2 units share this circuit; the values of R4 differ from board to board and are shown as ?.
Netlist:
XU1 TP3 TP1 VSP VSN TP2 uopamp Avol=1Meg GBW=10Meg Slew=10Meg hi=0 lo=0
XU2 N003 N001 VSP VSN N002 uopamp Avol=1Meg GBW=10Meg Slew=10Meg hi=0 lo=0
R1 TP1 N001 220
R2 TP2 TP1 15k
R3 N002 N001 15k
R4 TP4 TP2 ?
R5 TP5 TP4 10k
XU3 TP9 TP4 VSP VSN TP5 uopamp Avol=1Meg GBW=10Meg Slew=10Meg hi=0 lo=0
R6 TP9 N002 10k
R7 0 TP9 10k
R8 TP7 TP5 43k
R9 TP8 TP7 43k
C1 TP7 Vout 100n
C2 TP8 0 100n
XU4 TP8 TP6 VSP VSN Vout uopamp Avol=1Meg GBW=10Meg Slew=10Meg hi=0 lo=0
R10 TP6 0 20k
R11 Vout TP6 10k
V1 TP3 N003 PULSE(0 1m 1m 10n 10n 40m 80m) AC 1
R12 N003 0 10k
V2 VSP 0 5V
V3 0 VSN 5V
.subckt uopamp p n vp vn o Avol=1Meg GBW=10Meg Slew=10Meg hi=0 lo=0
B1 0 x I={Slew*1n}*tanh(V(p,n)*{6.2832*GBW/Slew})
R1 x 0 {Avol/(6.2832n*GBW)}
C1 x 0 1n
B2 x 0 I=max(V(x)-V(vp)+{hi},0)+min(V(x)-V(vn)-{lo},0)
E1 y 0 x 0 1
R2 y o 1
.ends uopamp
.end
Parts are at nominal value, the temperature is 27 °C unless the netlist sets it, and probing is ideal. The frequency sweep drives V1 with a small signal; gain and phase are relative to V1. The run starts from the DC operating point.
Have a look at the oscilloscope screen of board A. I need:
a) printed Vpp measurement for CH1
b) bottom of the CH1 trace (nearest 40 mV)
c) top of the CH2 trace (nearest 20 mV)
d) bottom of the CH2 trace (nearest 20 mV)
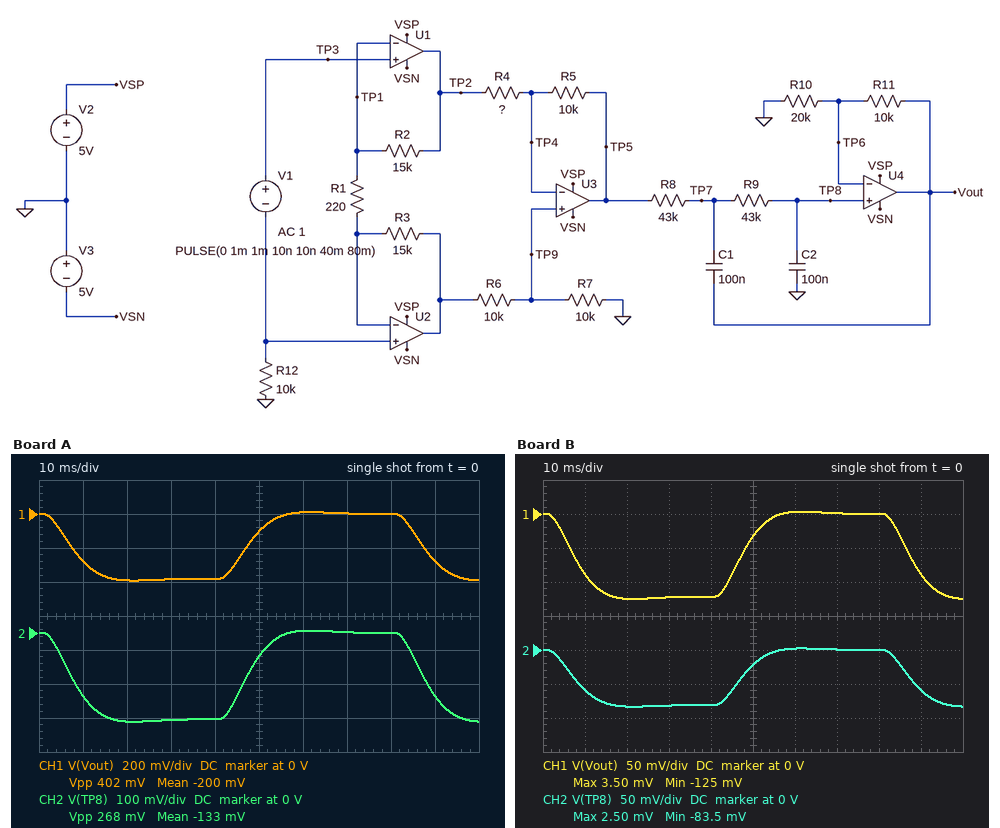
402 mV
-400 mV
0 V
-260 mV
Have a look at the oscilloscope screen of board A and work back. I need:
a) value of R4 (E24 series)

4.7 kΩ
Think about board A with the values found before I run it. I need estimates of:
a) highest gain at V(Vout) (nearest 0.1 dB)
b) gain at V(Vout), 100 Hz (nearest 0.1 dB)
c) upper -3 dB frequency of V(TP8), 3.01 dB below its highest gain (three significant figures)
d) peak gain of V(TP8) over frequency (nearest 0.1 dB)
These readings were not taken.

51.6 dB
34.1 dB
34.8 Hz
48.1 dB
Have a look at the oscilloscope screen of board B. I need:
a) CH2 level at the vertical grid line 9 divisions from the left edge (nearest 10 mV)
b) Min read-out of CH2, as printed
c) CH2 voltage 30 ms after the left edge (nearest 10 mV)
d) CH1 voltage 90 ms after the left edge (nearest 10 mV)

-60 mV
-83.5 mV
-80 mV
-90 mV
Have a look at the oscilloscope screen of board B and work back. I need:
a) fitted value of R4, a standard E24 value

22 kΩ
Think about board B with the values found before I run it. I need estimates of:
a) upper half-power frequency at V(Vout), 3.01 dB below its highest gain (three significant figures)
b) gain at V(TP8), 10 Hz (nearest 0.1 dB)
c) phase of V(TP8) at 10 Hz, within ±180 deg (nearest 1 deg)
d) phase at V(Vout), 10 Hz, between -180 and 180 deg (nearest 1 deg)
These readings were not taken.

34.8 Hz
38.1 dB
156 deg
156 deg
